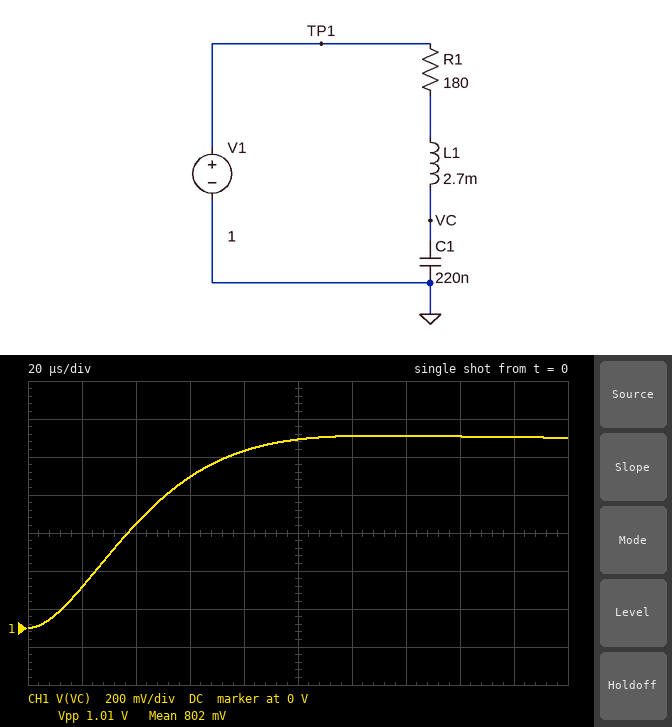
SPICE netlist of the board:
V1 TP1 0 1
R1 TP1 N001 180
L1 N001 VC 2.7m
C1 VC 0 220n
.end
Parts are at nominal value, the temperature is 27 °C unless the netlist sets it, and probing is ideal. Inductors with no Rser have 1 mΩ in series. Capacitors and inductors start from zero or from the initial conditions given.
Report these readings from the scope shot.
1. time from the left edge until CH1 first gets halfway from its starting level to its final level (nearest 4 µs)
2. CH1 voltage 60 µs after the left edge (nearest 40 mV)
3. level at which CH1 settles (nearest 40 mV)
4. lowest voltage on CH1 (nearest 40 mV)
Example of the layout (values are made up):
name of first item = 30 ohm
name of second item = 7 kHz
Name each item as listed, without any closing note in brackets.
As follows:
time from the left edge until CH1 first gets halfway from its starting level to its final level = 36 µs
CH1 voltage 60 µs after the left edge = 800 mV
level at which CH1 settles = 1.00 V
lowest voltage on CH1 = 0 V
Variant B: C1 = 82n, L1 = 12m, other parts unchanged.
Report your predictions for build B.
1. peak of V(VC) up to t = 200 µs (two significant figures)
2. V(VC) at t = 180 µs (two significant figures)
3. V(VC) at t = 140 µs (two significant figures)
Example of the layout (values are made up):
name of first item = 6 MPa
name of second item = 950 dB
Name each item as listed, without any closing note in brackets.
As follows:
peak of V(VC) up to t = 200 µs = 1.5 V
V(VC) at t = 180 µs = 840 mV
V(VC) at t = 140 µs = 1.2 V
